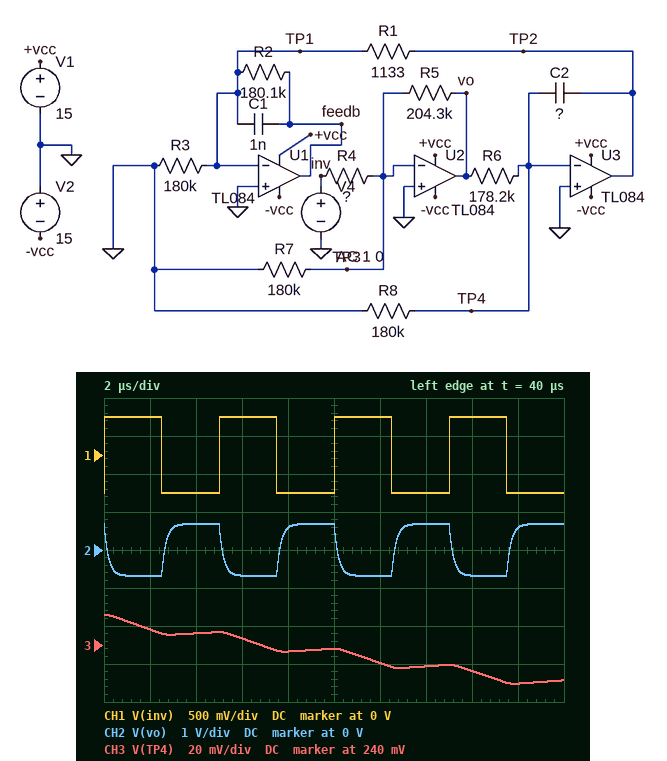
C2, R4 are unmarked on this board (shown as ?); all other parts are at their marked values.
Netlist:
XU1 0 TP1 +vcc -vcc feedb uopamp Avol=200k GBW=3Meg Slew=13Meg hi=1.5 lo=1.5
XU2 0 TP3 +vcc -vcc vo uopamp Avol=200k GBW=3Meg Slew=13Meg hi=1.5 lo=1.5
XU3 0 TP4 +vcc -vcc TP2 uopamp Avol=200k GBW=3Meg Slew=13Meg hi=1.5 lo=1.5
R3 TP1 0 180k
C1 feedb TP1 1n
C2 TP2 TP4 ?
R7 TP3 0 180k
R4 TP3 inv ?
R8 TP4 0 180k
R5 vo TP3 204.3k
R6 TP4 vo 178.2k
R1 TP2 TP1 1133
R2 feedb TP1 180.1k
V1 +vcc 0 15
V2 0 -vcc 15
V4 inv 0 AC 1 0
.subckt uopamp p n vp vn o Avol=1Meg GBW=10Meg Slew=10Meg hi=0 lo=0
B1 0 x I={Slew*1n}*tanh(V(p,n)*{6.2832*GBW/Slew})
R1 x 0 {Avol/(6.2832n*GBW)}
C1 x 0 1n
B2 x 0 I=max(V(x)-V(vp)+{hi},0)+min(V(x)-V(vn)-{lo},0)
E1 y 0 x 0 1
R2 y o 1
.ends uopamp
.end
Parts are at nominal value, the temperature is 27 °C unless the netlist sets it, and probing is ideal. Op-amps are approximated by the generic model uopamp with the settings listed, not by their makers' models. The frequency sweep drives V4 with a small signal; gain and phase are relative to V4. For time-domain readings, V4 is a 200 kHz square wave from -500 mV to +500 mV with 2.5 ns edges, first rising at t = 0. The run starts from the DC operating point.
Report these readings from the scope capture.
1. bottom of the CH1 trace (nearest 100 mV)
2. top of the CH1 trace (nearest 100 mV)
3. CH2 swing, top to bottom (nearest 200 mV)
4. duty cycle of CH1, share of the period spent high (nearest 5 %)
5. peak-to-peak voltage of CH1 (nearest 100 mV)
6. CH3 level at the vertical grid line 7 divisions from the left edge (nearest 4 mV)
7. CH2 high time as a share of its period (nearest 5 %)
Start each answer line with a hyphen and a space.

- -500 mV
- 500 mV
- 1.4 V
- 50 %
- 1.0 V
- 228 mV
- 50 %
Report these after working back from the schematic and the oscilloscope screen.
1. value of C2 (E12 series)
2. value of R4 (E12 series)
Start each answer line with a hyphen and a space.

- 1.5 nF
- 150 kΩ
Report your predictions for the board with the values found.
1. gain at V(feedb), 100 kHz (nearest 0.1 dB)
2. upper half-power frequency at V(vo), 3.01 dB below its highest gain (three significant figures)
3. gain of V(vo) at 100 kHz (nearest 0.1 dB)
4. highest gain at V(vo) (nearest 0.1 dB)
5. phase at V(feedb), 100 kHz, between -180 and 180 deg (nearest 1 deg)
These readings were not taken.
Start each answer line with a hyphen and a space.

- -39.3 dB
- 858 kHz
- 2.6 dB
- 2.7 dB
- -10 deg
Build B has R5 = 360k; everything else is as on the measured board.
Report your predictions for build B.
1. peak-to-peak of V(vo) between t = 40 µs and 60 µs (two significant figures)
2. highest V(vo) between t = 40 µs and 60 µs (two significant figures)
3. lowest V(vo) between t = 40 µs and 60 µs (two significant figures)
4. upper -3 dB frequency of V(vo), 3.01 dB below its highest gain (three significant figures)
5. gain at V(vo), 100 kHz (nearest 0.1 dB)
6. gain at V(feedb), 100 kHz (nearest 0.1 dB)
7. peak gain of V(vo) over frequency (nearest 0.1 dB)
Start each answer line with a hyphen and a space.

- 2.4 V
- 1.2 V
- -1.2 V
- 556 kHz
- 7.5 dB
- -34.5 dB
- 7.6 dB
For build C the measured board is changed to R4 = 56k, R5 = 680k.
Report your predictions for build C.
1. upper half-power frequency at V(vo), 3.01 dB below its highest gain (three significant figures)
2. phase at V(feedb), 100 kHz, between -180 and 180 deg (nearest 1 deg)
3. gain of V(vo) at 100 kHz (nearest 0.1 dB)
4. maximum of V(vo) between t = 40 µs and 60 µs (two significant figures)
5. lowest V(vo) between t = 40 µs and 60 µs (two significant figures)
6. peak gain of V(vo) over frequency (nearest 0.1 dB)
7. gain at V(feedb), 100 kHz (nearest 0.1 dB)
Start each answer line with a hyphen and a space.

- 177 kHz
- -33 deg
- 20.5 dB
- 5.3 V
- -5.3 V
- 21.7 dB
- -21.5 dB
